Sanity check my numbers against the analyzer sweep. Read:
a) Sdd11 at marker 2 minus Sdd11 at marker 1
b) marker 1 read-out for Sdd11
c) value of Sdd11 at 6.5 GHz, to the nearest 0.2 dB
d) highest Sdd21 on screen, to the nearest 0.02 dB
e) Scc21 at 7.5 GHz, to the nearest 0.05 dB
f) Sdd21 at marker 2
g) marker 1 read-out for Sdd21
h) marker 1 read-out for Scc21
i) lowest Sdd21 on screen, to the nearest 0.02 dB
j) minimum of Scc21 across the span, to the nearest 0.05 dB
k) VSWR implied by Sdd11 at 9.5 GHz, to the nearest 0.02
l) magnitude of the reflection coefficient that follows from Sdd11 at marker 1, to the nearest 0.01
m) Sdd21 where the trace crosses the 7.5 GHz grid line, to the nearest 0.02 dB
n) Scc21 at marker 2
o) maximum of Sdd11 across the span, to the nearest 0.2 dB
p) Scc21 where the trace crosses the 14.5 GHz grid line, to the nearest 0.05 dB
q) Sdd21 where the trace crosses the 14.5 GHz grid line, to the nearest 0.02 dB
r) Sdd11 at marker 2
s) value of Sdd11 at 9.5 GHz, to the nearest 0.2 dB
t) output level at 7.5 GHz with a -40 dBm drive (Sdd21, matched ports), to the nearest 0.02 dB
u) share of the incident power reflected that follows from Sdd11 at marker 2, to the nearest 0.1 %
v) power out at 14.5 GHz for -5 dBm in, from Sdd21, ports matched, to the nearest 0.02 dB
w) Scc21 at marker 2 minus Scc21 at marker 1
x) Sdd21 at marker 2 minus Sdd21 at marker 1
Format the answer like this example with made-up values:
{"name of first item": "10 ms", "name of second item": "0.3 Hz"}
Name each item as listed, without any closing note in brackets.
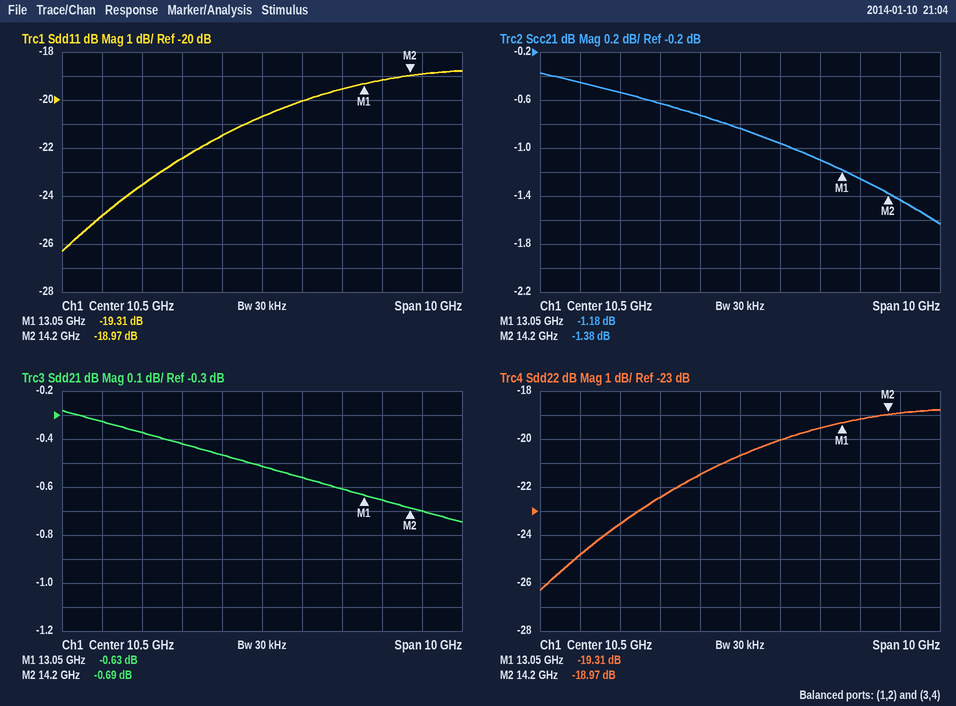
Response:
{"Sdd11 at marker 2 minus Sdd11 at marker 1": "0.34 dB", "marker 1 read-out for Sdd11": "-19.31 dB", "value of Sdd11 at 6.5 GHz, to the nearest 0.2 dB": "-24.8 dB", "highest Sdd21 on screen, to the nearest 0.02 dB": "-0.28 dB", "Scc21 at 7.5 GHz, to the nearest 0.05 dB": "-0.55 dB", "Sdd21 at marker 2": "-0.69 dB", "marker 1 read-out for Sdd21": "-0.63 dB", "marker 1 read-out for Scc21": "-1.18 dB", "lowest Sdd21 on screen, to the nearest 0.02 dB": "-0.74 dB", "minimum of Scc21 across the span, to the nearest 0.05 dB": "-1.65 dB", "VSWR implied by Sdd11 at 9.5 GHz, to the nearest 0.02": "1.18", "magnitude of the reflection coefficient that follows from Sdd11 at marker 1, to the nearest 0.01": "0.11", "Sdd21 where the trace crosses the 7.5 GHz grid line, to the nearest 0.02 dB": "-0.38 dB", "Scc21 at marker 2": "-1.38 dB", "maximum of Sdd11 across the span, to the nearest 0.2 dB": "-18.8 dB", "Scc21 where the trace crosses the 14.5 GHz grid line, to the nearest 0.05 dB": "-1.45 dB", "Sdd21 where the trace crosses the 14.5 GHz grid line, to the nearest 0.02 dB": "-0.70 dB", "Sdd11 at marker 2": "-18.97 dB", "value of Sdd11 at 9.5 GHz, to the nearest 0.2 dB": "-21.4 dB", "output level at 7.5 GHz with a -40 dBm drive (Sdd21, matched ports), to the nearest 0.02 dB": "-40.38 dBm", "share of the incident power reflected that follows from Sdd11 at marker 2, to the nearest 0.1 %": "1.3 %", "power out at 14.5 GHz for -5 dBm in, from Sdd21, ports matched, to the nearest 0.02 dB": "-5.70 dBm", "Scc21 at marker 2 minus Scc21 at marker 1": "-0.20 dB", "Sdd21 at marker 2 minus Sdd21 at marker 1": "-0.06 dB"}
